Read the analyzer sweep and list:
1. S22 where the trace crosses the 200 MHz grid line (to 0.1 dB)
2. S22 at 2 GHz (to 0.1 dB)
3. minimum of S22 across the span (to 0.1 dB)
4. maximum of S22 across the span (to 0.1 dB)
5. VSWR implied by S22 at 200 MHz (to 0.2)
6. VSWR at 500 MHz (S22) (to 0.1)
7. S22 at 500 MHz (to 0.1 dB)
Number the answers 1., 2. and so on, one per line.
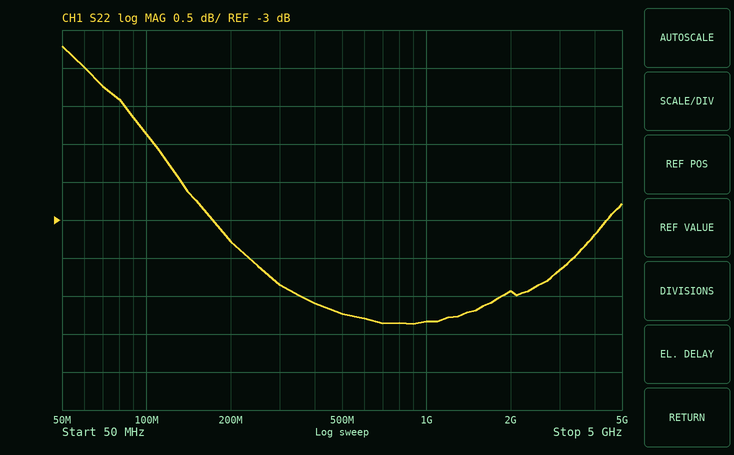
1. -3.3 dB
2. -3.9 dB
3. -4.4 dB
4. -0.7 dB
5. 5.4
6. 4.2
7. -4.2 dB
